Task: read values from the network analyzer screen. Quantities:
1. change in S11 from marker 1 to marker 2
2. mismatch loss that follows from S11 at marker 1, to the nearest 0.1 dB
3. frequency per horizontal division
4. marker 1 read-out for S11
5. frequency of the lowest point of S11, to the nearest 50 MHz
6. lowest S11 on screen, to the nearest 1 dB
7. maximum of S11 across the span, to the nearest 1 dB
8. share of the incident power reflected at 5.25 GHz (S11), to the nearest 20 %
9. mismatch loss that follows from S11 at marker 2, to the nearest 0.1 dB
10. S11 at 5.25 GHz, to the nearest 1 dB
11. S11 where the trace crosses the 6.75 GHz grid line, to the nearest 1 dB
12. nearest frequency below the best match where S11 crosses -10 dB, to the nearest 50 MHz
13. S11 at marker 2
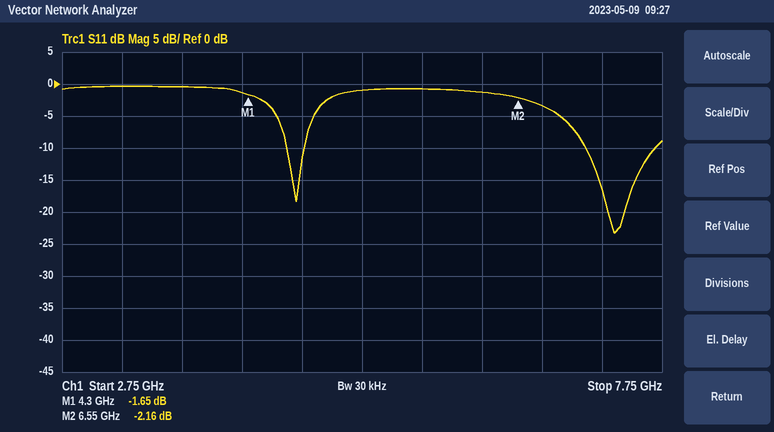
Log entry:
-0.51 dB
5.0 dB
500 MHz
-1.65 dB
7.35 GHz
-23 dB
0 dB
80 %
4.1 dB
-1 dB
-3 dB
7.10 GHz
-2.16 dB
